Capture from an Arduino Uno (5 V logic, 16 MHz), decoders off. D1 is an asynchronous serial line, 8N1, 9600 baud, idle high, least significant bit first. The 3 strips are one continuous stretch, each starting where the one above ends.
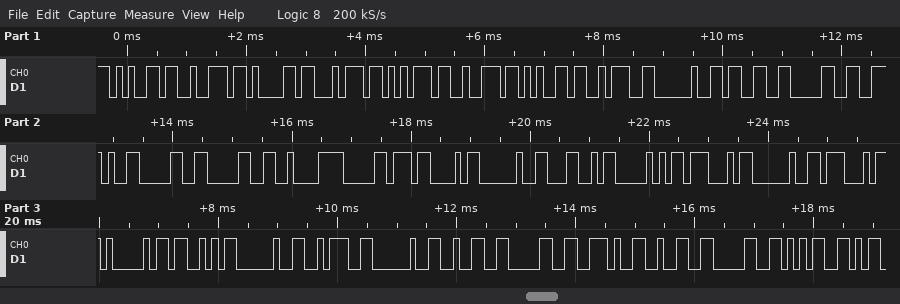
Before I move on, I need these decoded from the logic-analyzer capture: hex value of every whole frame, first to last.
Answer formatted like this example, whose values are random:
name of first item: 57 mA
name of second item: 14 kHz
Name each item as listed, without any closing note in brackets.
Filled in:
hex value of every whole frame, first to last: 65 72 61 74 75 72 65 3A 20 33 30 2E 30 30 C2 B0 43 20 4C 50 47 20 47 41 53 20 3A 20 32 30 2E 32 30 35
